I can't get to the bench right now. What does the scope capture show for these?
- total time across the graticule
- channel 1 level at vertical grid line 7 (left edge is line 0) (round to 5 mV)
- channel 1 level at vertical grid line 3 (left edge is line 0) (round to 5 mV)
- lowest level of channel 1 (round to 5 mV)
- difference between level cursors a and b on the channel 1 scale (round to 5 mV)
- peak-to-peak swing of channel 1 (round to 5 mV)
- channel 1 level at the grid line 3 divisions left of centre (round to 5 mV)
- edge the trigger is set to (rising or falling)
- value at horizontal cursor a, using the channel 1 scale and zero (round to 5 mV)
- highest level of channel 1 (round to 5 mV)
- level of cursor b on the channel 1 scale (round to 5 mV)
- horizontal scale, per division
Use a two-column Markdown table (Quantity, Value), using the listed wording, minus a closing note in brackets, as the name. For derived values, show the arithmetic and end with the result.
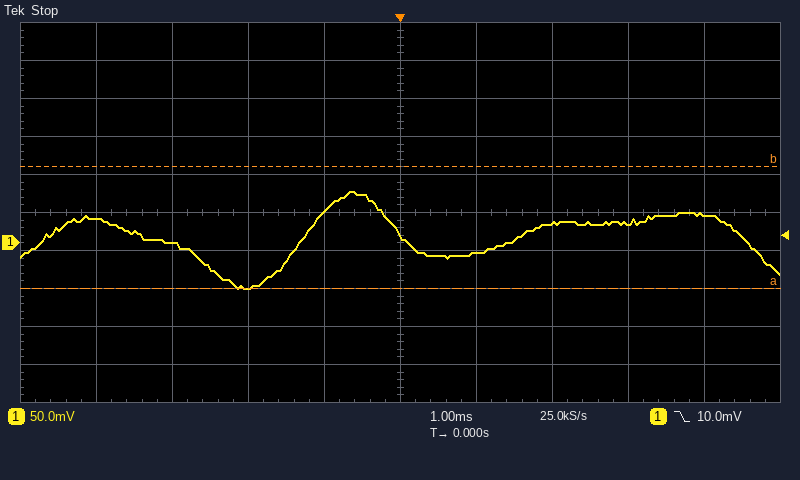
| Quantity | Value |
|---|---|
| total time across the graticule | 10 ms |
| channel 1 level at vertical grid line 7 (left edge is line 0) | 25 mV |
| channel 1 level at vertical grid line 3 (left edge is line 0) | -60 mV |
| lowest level of channel 1 | -60 mV |
| difference between level cursors a and b on the channel 1 scale | 160 mV |
| peak-to-peak swing of channel 1 | 70 mV − (-60 mV) = 130 mV |
| channel 1 level at the grid line 3 divisions left of centre | 0 mV |
| edge the trigger is set to | falling |
| value at horizontal cursor a, using the channel 1 scale and zero | -60 mV |
| highest level of channel 1 | 70 mV |
| level of cursor b on the channel 1 scale | 100 mV |
| horizontal scale, per division | 1 ms |
